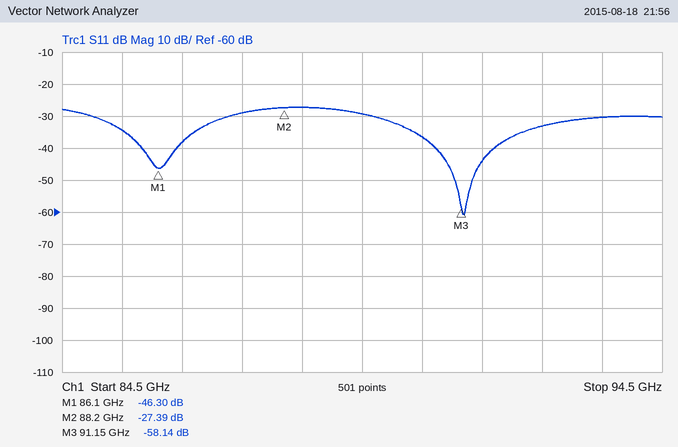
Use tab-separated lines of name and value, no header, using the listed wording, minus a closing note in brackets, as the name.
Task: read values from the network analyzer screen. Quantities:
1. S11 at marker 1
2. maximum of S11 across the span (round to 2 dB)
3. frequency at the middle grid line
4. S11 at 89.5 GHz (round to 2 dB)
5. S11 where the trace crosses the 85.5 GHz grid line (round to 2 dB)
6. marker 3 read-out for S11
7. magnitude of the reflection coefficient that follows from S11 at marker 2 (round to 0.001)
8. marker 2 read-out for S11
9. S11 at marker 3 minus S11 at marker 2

S11 at marker 1	-46.30 dB
maximum of S11 across the span	-28 dB
frequency at the middle grid line	89.5 GHz
S11 at 89.5 GHz	-30 dB
S11 where the trace crosses the 85.5 GHz grid line	-34 dB
marker 3 read-out for S11	-58.14 dB
magnitude of the reflection coefficient that follows from S11 at marker 2	0.043
marker 2 read-out for S11	-27.39 dB
S11 at marker 3 minus S11 at marker 2	-30.75 dB
